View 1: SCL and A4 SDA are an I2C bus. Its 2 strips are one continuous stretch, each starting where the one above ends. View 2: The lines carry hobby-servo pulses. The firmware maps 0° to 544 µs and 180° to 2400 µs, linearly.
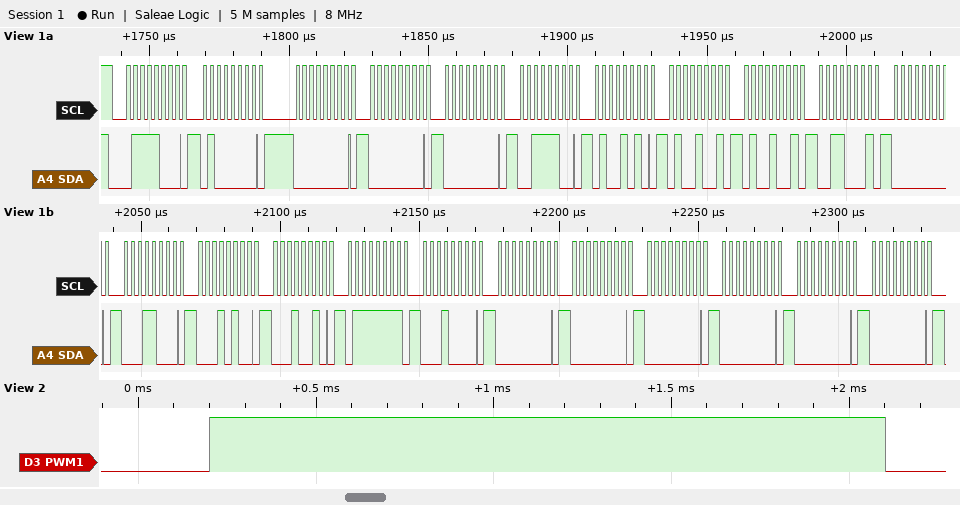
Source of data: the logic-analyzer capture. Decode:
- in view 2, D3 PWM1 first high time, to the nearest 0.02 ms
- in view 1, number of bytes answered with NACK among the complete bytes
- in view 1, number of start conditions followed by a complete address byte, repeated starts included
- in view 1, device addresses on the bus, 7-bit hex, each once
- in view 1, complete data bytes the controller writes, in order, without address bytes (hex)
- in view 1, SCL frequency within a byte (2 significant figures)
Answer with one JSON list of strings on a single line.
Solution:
["1.90 ms", "0", "1", "0x3C", "40 00 00 00 3C 4A 49 49 31 00 18 14 12 7F 10 00 00 00 00 00 00", "400 kHz"]
